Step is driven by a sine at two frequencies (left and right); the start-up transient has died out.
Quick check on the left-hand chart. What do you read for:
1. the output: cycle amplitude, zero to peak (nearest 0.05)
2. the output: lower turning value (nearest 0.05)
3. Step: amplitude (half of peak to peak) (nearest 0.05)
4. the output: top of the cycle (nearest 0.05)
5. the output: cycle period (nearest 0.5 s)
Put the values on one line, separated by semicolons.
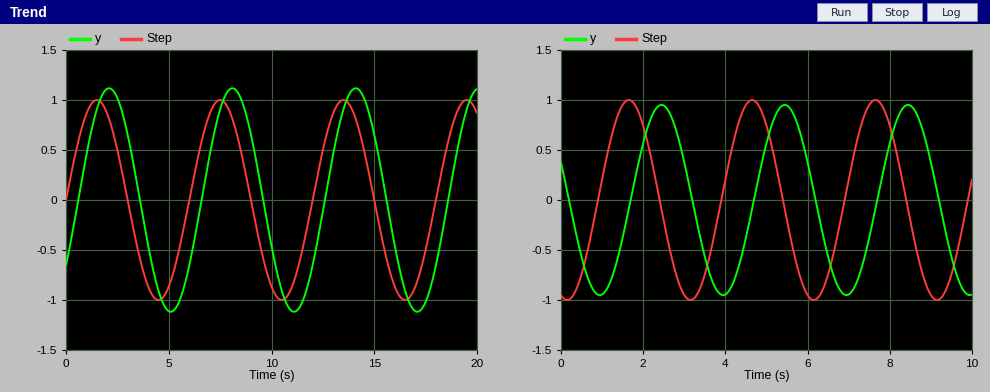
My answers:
1.10; -1.10; 1.00; 1.10; 6.0 s
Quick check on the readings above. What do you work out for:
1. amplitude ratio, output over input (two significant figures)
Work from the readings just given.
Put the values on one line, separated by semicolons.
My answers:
1.1
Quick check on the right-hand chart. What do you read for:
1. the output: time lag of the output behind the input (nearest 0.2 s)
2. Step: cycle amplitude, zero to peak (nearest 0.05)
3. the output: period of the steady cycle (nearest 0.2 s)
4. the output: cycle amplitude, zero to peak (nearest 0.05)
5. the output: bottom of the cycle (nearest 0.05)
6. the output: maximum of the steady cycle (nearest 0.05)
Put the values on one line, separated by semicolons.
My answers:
0.8 s; 1.00; 3.0 s; 0.95; -0.95; 0.95
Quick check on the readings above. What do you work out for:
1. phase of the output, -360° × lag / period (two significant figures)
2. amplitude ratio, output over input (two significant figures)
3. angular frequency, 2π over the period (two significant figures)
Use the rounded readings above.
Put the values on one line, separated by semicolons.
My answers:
-96°; 0.95; 2.1 rad/s
